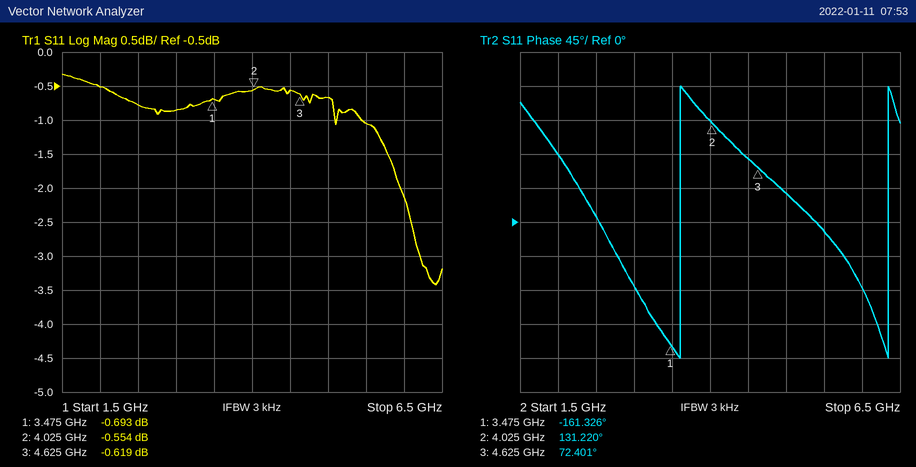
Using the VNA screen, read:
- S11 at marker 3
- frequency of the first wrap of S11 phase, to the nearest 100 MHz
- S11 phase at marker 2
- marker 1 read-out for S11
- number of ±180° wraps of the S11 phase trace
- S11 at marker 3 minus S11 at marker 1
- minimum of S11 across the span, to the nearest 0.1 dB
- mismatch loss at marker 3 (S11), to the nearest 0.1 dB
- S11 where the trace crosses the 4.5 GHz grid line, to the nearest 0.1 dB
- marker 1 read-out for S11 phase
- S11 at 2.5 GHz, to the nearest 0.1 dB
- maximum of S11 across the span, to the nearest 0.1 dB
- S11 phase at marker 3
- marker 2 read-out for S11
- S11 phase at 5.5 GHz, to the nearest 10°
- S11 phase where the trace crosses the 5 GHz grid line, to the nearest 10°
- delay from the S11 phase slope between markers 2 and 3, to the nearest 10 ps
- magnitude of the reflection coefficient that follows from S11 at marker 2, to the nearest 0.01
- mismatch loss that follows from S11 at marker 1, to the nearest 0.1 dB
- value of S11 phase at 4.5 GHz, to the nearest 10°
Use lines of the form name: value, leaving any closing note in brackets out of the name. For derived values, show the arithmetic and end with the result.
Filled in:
S11 at marker 3: -0.619 dB
frequency of the first wrap of S11 phase, to the nearest 100 MHz: 3.6 GHz
S11 phase at marker 2: 131.220°
marker 1 read-out for S11: -0.693 dB
number of ±180° wraps of the S11 phase trace: 2
S11 at marker 3 minus S11 at marker 1: -0.619 − (-0.693) = 0.074 dB
minimum of S11 across the span, to the nearest 0.1 dB: -3.4 dB
mismatch loss at marker 3 (S11), to the nearest 0.1 dB: −10 log10(1 − 10^(-0.619/10)) ≈ 8.8 dB
S11 where the trace crosses the 4.5 GHz grid line, to the nearest 0.1 dB: -0.6 dB
marker 1 read-out for S11 phase: -161.326°
S11 at 2.5 GHz, to the nearest 0.1 dB: -0.8 dB
maximum of S11 across the span, to the nearest 0.1 dB: -0.3 dB
S11 phase at marker 3: 72.401°
marker 2 read-out for S11: -0.554 dB
S11 phase at 5.5 GHz, to the nearest 10°: -10°
S11 phase where the trace crosses the 5 GHz grid line, to the nearest 10°: 40°
delay from the S11 phase slope between markers 2 and 3, to the nearest 10 ps: −(72.401° − (131.22°))/(360° × 600 MHz) ≈ 272 ps, so 270 ps to the nearest 10 ps
magnitude of the reflection coefficient that follows from S11 at marker 2, to the nearest 0.01: 10^(-0.554/20) ≈ 0.94
mismatch loss that follows from S11 at marker 1, to the nearest 0.1 dB: −10 log10(1 − 10^(-0.693/10)) ≈ 8.3 dB
value of S11 phase at 4.5 GHz, to the nearest 10°: 80°
